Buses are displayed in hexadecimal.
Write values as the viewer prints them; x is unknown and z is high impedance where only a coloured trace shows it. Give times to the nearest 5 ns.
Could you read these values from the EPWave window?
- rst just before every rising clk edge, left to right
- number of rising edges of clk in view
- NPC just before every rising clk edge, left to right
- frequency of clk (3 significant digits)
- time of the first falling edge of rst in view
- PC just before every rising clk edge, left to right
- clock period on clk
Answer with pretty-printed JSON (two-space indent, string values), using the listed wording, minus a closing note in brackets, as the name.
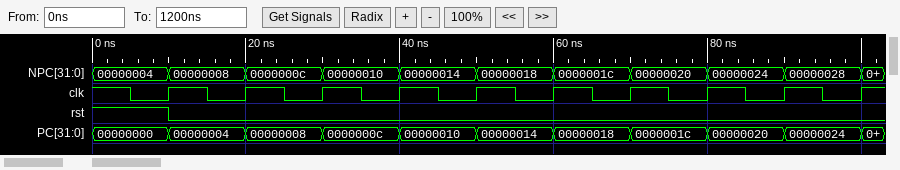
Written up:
{
  "rst just before every rising clk edge, left to right": "1 0 0 0 0 0 0 0 0 0",
  "number of rising edges of clk in view": "10",
  "NPC just before every rising clk edge, left to right": "00000004, 00000008, 0000000c, 00000010, 00000014, 00000018, 0000001c, 00000020, 00000024, 00000028",
  "frequency of clk": "100 MHz",
  "time of the first falling edge of rst in view": "10 ns",
  "PC just before every rising clk edge, left to right": "00000000, 00000004, 00000008, 0000000c, 00000010, 00000014, 00000018, 0000001c, 00000020, 00000024",
  "clock period on clk": "10 ns"
}
